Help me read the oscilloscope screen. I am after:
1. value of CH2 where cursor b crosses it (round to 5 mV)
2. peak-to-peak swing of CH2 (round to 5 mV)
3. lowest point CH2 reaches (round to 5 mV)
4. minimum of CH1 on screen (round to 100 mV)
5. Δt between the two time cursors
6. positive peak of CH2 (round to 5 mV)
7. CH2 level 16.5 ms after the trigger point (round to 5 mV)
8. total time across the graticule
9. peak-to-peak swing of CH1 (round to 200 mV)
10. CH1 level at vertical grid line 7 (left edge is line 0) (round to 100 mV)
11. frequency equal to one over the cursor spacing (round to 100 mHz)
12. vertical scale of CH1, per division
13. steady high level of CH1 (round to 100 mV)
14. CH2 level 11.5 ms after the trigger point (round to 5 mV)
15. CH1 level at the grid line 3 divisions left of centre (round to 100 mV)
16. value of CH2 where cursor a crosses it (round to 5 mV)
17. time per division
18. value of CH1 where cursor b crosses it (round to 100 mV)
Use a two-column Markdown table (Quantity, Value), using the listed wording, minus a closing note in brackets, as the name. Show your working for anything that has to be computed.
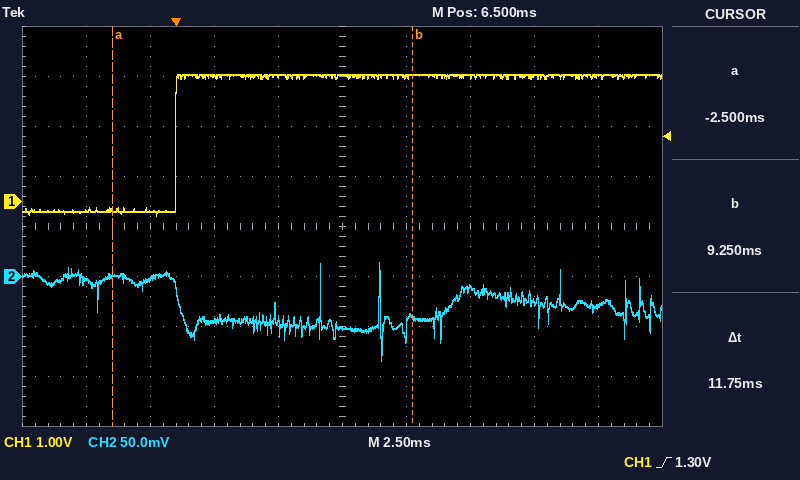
| Quantity | Value |
|---|---|
| value of CH2 where cursor b crosses it | -40 mV |
| peak-to-peak swing of CH2 | 15 mV − (-85 mV) = 100 mV |
| lowest point CH2 reaches | -85 mV |
| minimum of CH1 on screen | -300 mV |
| Δt between the two time cursors | 11.75 ms |
| positive peak of CH2 | 15 mV |
| CH2 level 16.5 ms after the trigger point | -30 mV |
| total time across the graticule | 25 ms |
| peak-to-peak swing of CH1 | 2.8 V |
| CH1 level at vertical grid line 7 (left edge is line 0) | 2.5 V |
| frequency equal to one over the cursor spacing | 1 / 11.75 ms ≈ 85.1 Hz |
| vertical scale of CH1, per division | 1 V |
| steady high level of CH1 | 2.5 V |
| CH2 level 11.5 ms after the trigger point | -10 mV |
| CH1 level at the grid line 3 divisions left of centre | -200 mV |
| value of CH2 where cursor a crosses it | 0 mV |
| time per division | 2.5 ms |
| value of CH1 where cursor b crosses it | 2.5 V |
